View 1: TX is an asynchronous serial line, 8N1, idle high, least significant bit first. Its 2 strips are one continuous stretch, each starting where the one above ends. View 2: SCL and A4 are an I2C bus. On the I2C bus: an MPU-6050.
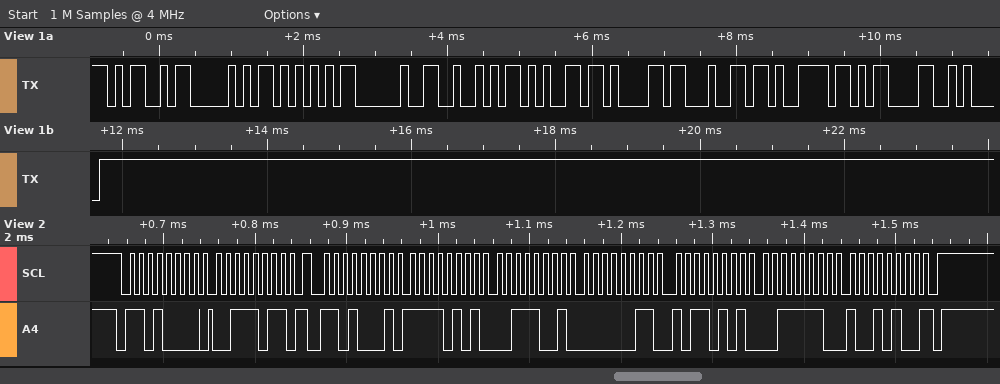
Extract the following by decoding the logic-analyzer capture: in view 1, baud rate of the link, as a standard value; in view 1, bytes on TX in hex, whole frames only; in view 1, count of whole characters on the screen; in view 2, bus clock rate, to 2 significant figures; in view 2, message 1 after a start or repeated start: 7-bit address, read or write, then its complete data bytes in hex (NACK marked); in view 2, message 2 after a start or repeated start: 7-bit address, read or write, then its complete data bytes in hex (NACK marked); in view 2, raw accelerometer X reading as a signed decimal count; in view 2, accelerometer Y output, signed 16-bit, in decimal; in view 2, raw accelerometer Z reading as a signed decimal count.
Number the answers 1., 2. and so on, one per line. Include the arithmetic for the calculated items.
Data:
1. 9600 baud
2. 4D 50 55 20 52 65 61 64 79 0D 0A
3. 11
4. 100 kHz
5. 0x68 write: 3B
6. 0x68 read: F5 39 03 B5 3E 94 NACK
7. 0xF539 = -2759
8. 0x03B5 = 949
9. 0x3E94 = 16020
